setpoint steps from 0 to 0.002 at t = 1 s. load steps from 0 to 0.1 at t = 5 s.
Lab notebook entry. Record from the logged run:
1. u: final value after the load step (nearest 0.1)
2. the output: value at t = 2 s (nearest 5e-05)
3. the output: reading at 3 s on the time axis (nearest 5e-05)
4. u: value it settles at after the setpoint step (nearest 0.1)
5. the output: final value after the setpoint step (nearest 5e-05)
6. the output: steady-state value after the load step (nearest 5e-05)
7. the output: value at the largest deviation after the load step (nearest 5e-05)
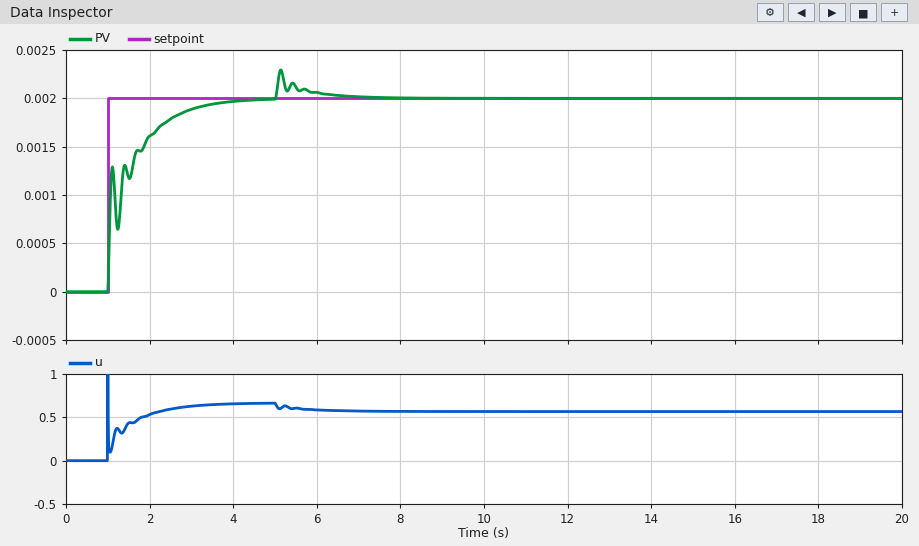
0.6
0.00160
0.00190
0.7
0.00200
0.00200
0.00230
